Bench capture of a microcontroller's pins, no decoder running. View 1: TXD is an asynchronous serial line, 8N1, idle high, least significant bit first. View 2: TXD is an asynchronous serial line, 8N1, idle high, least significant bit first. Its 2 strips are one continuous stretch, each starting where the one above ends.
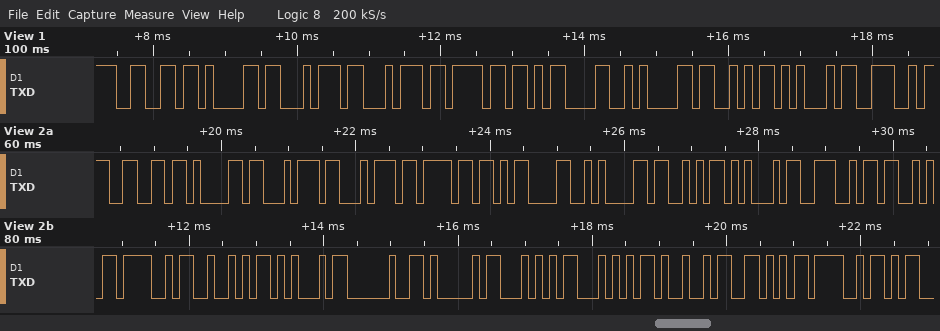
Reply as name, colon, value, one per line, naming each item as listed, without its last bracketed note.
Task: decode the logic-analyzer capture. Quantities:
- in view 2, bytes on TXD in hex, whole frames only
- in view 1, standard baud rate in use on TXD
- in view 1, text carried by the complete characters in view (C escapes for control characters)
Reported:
in view 2, bytes on TXD in hex, whole frames only: 66 61 74 74 6F 0D 0A 53 45 4E 53 4F 52 45 20 41 54 54 49 56 4F
in view 1, standard baud rate in use on TXD: 9600 baud
in view 1, text carried by the complete characters in view: "fatto\r\nSEN"
